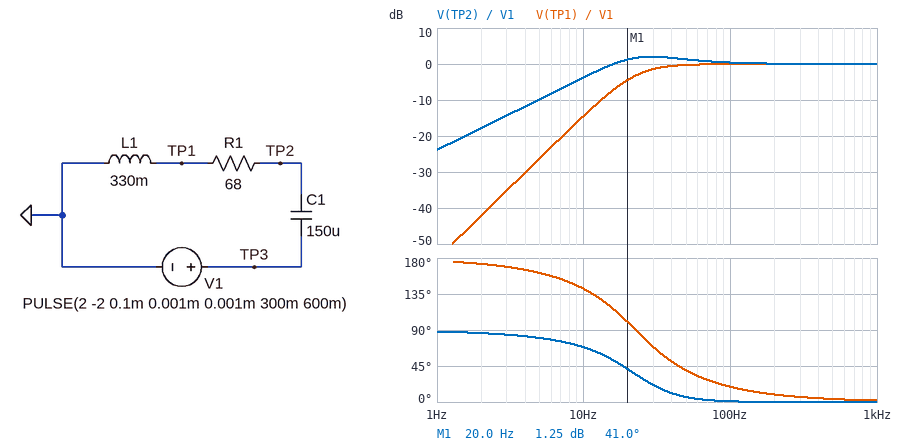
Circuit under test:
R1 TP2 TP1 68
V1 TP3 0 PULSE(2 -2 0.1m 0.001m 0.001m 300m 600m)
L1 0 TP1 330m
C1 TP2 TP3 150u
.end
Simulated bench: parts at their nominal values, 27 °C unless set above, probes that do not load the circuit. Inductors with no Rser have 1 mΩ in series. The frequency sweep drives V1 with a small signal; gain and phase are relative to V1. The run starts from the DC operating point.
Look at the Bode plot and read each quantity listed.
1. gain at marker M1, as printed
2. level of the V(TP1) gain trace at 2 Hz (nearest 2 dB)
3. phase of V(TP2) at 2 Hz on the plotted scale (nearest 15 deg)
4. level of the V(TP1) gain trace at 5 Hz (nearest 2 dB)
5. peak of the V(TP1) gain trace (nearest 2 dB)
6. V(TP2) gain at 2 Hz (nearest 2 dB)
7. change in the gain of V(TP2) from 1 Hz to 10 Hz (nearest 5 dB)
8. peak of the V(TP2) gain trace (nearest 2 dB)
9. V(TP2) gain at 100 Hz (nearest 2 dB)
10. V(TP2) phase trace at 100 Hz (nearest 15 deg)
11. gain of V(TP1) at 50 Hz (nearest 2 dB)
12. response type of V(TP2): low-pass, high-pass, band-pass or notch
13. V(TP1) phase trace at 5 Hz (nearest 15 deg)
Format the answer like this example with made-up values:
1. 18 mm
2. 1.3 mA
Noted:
1. 1.25 dB
2. -42 dB
3. 90 deg
4. -26 dB
5. 0 dB
6. -18 dB
7. 20 dB
8. 2 dB
9. 0 dB
10. 0 deg
11. 0 dB
12. high-pass
13. 165 deg
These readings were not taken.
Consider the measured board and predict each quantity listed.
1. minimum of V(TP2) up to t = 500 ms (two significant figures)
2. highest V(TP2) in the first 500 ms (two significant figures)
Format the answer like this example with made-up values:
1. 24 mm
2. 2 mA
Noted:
1. -4.0 V
2. 4.0 V
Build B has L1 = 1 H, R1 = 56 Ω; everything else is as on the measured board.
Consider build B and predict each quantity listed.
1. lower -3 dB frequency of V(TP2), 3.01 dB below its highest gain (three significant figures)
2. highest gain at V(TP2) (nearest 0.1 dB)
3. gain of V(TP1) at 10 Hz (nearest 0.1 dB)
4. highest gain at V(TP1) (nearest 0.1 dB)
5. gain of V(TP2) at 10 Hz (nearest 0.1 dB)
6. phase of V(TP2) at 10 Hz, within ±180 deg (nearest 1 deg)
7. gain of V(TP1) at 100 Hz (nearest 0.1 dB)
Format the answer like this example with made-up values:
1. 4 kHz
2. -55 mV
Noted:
1. 10.4 Hz
2. 5.2 dB
3. -1.0 dB
4. 3.8 dB
5. 1.5 dB
6. 86 deg
7. 0.1 dB
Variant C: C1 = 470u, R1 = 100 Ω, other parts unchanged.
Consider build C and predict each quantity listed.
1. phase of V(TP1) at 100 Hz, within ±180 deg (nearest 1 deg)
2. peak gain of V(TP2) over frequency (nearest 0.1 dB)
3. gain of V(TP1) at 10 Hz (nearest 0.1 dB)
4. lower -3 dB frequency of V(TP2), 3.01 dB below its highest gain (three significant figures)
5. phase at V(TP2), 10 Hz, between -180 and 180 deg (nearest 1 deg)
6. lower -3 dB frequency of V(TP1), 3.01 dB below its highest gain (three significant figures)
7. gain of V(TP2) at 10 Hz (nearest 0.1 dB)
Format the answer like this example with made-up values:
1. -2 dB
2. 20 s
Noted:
1. 26 deg
2. 0.4 dB
3. -13.7 dB
4. 3.47 Hz
5. 19 deg
6. 44.9 Hz
7. 0.1 dB
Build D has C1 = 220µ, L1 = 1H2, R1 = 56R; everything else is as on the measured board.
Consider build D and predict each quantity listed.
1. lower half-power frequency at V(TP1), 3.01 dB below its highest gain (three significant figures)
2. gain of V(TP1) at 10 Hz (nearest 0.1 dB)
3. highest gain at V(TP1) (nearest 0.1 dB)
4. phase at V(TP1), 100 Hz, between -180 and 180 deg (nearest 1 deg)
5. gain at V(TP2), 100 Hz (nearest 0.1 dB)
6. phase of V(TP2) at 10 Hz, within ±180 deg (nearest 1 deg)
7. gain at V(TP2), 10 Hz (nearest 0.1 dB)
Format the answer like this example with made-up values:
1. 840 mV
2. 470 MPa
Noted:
1. 8.24 Hz
2. 2.6 dB
3. 3.1 dB
4. 4 deg
5. 0.1 dB
6. 50 deg
7. 4.5 dB
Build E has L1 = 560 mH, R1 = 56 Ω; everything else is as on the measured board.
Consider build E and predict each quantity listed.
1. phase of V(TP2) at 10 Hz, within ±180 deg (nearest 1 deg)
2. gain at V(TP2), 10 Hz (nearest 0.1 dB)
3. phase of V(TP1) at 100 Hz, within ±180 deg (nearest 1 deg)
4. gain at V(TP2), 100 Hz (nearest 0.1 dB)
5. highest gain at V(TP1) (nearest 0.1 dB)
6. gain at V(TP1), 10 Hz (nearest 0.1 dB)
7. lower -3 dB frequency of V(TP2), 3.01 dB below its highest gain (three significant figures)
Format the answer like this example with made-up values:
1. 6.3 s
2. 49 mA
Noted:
1. 84 deg
2. -2.7 dB
3. 9 deg
4. 0.3 dB
5. 1.8 dB
6. -8.2 dB
7. 13.0 Hz
